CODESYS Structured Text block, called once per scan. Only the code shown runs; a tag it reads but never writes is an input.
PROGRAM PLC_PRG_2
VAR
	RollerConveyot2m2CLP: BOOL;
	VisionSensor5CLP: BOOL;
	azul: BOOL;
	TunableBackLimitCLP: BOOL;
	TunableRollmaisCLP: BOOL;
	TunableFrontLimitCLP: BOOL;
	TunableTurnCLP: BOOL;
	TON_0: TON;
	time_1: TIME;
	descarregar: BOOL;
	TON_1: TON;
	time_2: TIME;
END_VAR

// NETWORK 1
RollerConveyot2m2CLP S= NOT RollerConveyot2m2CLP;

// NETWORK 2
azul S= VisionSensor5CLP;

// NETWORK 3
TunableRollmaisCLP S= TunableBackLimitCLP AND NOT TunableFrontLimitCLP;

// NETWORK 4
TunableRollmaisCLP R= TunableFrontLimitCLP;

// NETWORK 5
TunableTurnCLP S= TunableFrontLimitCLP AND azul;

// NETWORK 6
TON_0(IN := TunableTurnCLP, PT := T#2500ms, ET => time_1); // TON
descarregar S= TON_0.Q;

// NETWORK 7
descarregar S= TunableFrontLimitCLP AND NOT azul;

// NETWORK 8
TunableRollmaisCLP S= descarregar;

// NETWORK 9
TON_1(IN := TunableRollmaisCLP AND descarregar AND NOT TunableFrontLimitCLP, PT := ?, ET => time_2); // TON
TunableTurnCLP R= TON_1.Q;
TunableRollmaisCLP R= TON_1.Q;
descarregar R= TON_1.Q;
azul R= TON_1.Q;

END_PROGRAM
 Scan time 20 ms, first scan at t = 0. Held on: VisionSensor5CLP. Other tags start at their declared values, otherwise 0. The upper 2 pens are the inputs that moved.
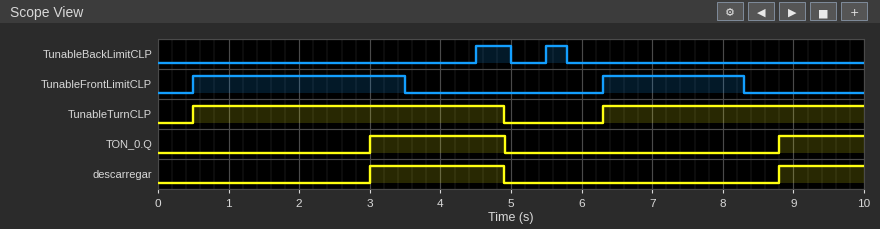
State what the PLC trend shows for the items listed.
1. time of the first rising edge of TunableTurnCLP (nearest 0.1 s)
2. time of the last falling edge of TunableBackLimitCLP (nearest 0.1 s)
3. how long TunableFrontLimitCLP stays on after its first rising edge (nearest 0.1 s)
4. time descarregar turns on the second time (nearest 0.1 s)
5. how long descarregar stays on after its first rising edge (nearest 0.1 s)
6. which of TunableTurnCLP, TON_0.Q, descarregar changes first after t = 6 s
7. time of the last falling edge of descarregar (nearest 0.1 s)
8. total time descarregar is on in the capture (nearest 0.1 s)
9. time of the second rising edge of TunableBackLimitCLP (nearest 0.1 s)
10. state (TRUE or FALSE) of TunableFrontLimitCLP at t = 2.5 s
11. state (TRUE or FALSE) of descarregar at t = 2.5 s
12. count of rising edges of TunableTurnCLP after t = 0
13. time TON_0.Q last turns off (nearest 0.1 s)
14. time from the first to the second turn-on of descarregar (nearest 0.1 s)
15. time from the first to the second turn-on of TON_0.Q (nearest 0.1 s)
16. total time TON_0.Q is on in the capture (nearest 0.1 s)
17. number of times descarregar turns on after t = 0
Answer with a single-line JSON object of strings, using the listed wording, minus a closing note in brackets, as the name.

{"time of the first rising edge of TunableTurnCLP": "0.5 s", "time of the last falling edge of TunableBackLimitCLP": "5.8 s", "how long TunableFrontLimitCLP stays on after its first rising edge": "3.0 s", "time descarregar turns on the second time": "8.8 s", "how long descarregar stays on after its first rising edge": "1.9 s", "which of TunableTurnCLP, TON_0.Q, descarregar changes first after t = 6 s": "TunableTurnCLP", "time of the last falling edge of descarregar": "4.9 s", "total time descarregar is on in the capture": "3.1 s", "time of the second rising edge of TunableBackLimitCLP": "5.5 s", "state (TRUE or FALSE) of TunableFrontLimitCLP at t = 2.5 s": "TRUE", "state (TRUE or FALSE) of descarregar at t = 2.5 s": "FALSE", "count of rising edges of TunableTurnCLP after t = 0": "2", "time TON_0.Q last turns off": "4.9 s", "time from the first to the second turn-on of descarregar": "5.8 s", "time from the first to the second turn-on of TON_0.Q": "5.8 s", "total time TON_0.Q is on in the capture": "3.1 s", "number of times descarregar turns on after t = 0": "2"}
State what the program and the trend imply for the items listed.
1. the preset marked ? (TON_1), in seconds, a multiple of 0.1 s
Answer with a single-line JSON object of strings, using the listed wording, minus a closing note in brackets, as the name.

{"the preset marked ? (TON_1), in seconds, a multiple of 0.1 s": "1.4 s"}
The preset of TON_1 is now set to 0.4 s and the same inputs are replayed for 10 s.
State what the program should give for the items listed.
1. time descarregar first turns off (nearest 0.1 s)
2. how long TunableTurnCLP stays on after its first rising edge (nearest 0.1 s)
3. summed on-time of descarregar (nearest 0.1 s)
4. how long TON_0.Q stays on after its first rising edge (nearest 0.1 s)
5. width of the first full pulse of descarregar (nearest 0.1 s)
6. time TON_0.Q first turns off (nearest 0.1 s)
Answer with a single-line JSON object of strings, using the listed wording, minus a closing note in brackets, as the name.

{"time descarregar first turns off": "3.9 s", "how long TunableTurnCLP stays on after its first rising edge": "3.4 s", "summed on-time of descarregar": "1.3 s", "how long TON_0.Q stays on after its first rising edge": "0.9 s", "width of the first full pulse of descarregar": "0.9 s", "time TON_0.Q first turns off": "3.9 s"}
